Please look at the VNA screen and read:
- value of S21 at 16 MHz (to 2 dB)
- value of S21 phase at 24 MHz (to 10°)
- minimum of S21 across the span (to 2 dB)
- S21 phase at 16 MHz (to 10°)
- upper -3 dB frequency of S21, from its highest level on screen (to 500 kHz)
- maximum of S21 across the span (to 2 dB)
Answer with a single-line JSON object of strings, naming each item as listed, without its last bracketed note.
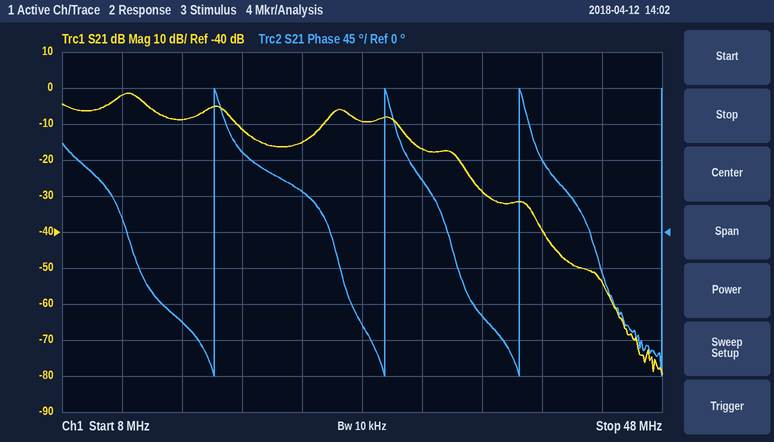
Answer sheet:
{"value of S21 at 16 MHz": "-8 dB", "value of S21 phase at 24 MHz": "50°", "minimum of S21 across the span": "-80 dB", "S21 phase at 16 MHz": "-110°", "upper -3 dB frequency of S21, from its highest level on screen": "13.5 MHz", "maximum of S21 across the span": "-2 dB"}
